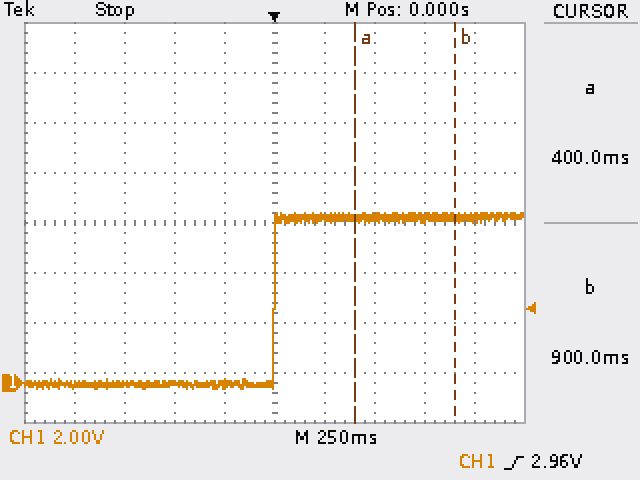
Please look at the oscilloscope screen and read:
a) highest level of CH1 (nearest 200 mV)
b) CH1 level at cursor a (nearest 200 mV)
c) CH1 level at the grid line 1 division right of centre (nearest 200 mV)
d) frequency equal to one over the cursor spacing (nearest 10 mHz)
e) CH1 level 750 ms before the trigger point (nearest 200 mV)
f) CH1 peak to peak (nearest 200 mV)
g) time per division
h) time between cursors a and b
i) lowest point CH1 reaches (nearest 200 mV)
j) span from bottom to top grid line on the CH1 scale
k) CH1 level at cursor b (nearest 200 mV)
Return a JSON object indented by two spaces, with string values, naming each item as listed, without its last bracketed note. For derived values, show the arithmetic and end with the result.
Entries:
{
  "highest level of CH1": "6.8 V",
  "CH1 level at cursor a": "6.6 V",
  "CH1 level at the grid line 1 division right of centre": "6.6 V",
  "frequency equal to one over the cursor spacing": "1 / 500 ms ≈ 2.00 Hz",
  "CH1 level 750 ms before the trigger point": "0.0 V",
  "CH1 peak to peak": "6.8 V − (-200 mV) = 7.0 V",
  "time per division": "250 ms",
  "time between cursors a and b": "900 ms − (400 ms) = 500 ms",
  "lowest point CH1 reaches": "-200 mV",
  "span from bottom to top grid line on the CH1 scale": "16 V",
  "CH1 level at cursor b": "6.6 V"
}
